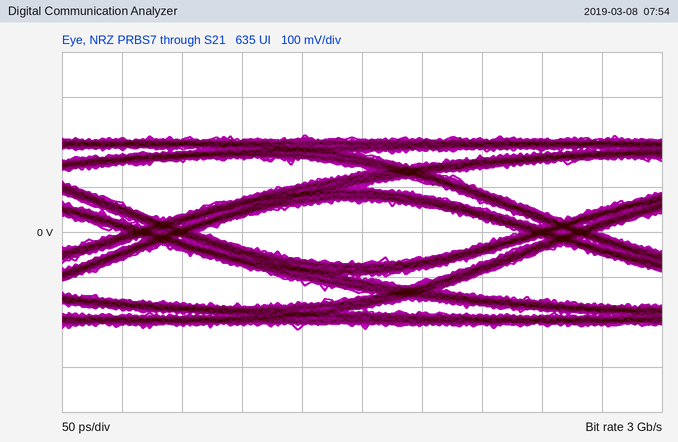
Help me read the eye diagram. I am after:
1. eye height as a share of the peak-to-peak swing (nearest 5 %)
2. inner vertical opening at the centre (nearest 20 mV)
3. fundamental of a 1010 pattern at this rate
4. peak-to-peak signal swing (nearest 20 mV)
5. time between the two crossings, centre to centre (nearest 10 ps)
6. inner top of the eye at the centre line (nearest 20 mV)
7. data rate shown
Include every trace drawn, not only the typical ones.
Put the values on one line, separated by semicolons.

30 %; 140 mV; 1.5 GHz; 440 mV; 330 ps; 60 mV; 3 Gb/s
